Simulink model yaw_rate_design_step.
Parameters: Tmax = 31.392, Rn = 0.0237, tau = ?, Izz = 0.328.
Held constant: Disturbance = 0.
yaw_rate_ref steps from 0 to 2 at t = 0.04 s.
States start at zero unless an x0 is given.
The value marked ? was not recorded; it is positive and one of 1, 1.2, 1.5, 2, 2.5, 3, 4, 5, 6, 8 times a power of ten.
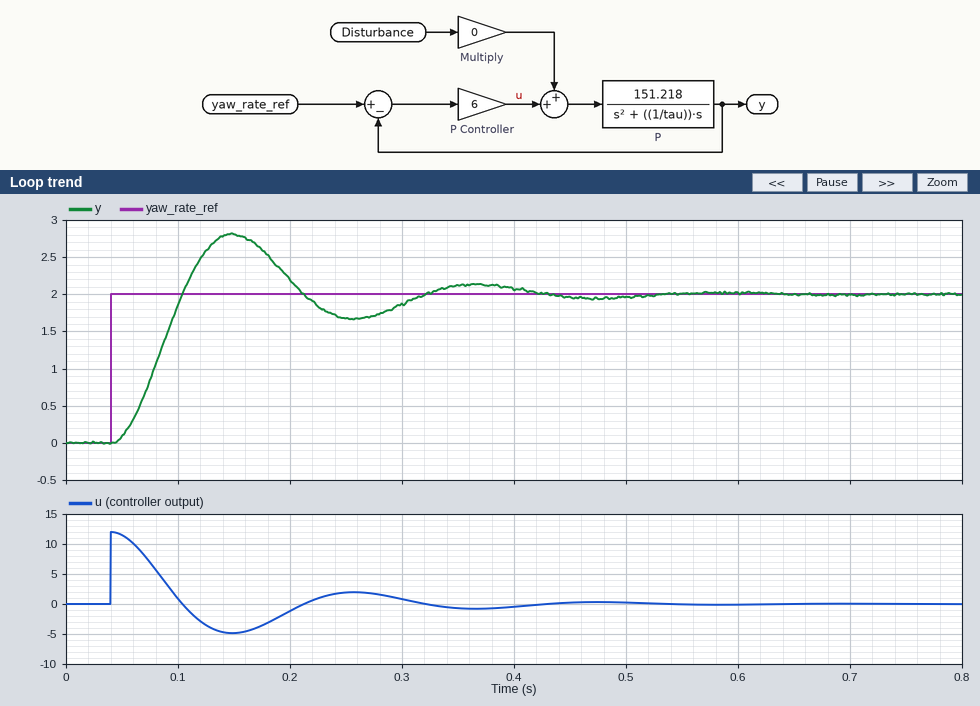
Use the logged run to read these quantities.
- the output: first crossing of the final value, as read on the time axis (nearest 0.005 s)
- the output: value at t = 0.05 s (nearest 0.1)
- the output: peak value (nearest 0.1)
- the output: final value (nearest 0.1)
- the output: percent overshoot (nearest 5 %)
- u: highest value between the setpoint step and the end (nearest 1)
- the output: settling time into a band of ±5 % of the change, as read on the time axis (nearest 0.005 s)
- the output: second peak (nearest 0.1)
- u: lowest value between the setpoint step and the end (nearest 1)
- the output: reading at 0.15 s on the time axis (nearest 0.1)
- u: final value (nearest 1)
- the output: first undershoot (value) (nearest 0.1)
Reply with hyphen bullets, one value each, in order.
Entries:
- 0.105 s
- 0.1
- 2.8
- 2.0
- 40 %
- 12
- 0.390 s
- 2.1
- -5
- 2.8
- 0
- 1.7
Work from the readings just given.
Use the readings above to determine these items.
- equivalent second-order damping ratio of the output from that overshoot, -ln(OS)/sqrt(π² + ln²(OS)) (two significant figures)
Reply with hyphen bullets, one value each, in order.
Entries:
- 0.28
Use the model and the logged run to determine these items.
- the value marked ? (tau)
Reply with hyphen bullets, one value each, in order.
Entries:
- 0.06
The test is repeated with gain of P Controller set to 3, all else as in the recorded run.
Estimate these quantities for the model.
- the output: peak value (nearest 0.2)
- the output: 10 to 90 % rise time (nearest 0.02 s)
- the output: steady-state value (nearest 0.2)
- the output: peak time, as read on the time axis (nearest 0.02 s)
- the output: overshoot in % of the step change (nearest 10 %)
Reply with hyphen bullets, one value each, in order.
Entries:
- 2.6
- 0.06 s
- 2.0
- 0.20 s
- 30 %
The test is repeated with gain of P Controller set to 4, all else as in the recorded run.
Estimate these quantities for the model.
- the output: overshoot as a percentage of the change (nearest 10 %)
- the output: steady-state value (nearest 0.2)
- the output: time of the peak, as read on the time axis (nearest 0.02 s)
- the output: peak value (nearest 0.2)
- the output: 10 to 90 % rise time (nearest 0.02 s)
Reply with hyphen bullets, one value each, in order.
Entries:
- 30 %
- 2.0
- 0.18 s
- 2.6
- 0.06 s
